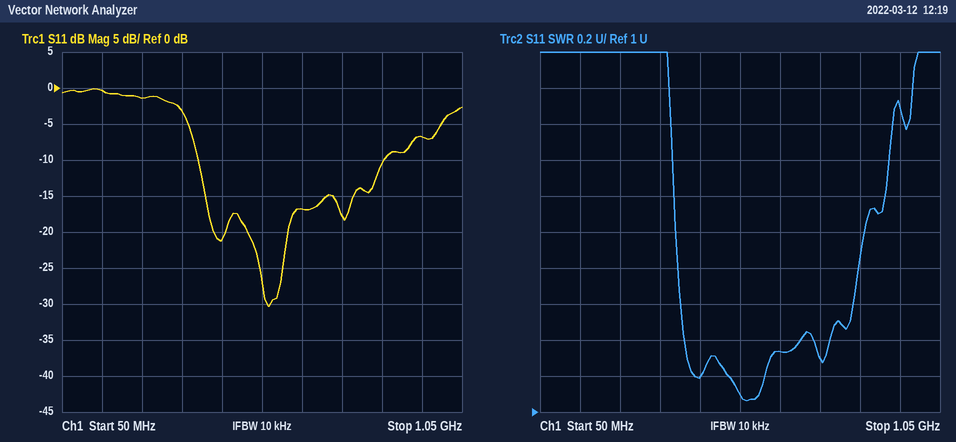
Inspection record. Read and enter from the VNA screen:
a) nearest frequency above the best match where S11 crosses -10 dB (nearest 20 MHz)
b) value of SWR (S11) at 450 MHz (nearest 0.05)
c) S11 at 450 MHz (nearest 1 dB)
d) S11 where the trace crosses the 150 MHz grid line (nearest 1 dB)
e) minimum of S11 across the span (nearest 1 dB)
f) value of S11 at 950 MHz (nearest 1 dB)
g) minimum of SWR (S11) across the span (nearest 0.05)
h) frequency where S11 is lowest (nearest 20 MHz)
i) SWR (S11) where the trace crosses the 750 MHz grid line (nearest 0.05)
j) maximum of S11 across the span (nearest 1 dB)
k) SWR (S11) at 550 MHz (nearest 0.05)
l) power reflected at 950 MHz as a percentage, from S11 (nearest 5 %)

860 MHz
1.20
-21 dB
0 dB
-30 dB
-7 dB
1.05
560 MHz
1.30
0 dB
1.10
20 %
